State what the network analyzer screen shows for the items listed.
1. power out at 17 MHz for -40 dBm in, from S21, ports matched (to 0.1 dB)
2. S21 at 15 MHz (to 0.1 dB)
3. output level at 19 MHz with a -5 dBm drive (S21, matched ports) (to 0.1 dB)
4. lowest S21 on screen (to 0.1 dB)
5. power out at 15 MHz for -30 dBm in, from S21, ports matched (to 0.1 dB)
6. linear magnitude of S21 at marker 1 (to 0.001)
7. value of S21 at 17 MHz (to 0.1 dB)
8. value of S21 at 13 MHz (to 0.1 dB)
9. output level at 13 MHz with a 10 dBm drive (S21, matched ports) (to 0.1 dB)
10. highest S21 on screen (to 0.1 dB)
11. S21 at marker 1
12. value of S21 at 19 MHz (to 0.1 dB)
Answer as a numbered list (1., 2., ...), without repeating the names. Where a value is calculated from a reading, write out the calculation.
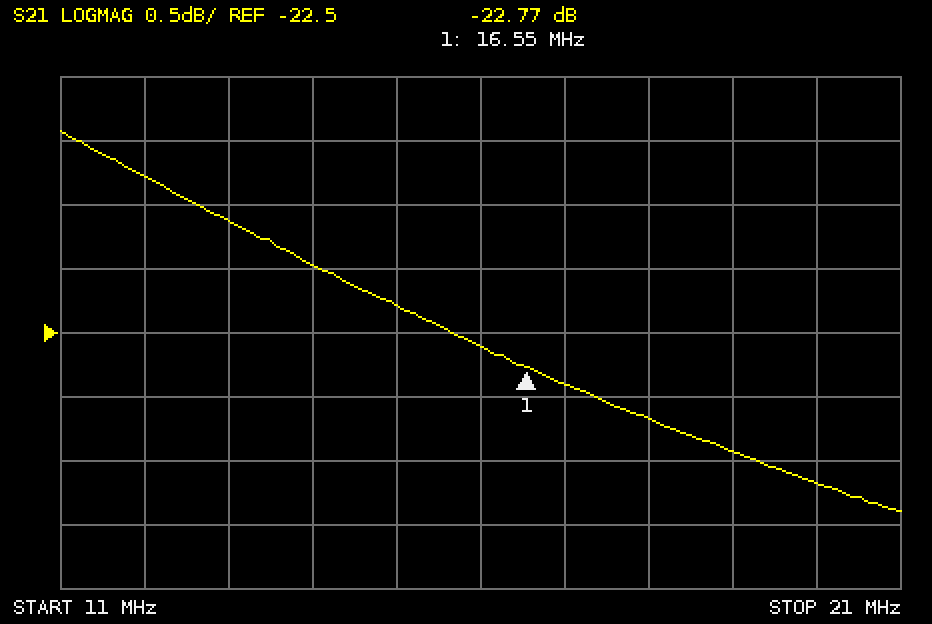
1. -40 dBm + (-22.9 dB) = -62.9 dBm
2. -22.3 dB
3. -5 dBm + (-23.4 dB) = -28.4 dBm
4. -23.9 dB
5. -30 dBm + (-22.3 dB) = -52.3 dBm
6. 10^(-22.77/20) ≈ 0.073
7. -22.9 dB
8. -21.6 dB
9. 10 dBm + (-21.6 dB) = -11.6 dBm
10. -20.9 dB
11. -22.77 dB
12. -23.4 dB
